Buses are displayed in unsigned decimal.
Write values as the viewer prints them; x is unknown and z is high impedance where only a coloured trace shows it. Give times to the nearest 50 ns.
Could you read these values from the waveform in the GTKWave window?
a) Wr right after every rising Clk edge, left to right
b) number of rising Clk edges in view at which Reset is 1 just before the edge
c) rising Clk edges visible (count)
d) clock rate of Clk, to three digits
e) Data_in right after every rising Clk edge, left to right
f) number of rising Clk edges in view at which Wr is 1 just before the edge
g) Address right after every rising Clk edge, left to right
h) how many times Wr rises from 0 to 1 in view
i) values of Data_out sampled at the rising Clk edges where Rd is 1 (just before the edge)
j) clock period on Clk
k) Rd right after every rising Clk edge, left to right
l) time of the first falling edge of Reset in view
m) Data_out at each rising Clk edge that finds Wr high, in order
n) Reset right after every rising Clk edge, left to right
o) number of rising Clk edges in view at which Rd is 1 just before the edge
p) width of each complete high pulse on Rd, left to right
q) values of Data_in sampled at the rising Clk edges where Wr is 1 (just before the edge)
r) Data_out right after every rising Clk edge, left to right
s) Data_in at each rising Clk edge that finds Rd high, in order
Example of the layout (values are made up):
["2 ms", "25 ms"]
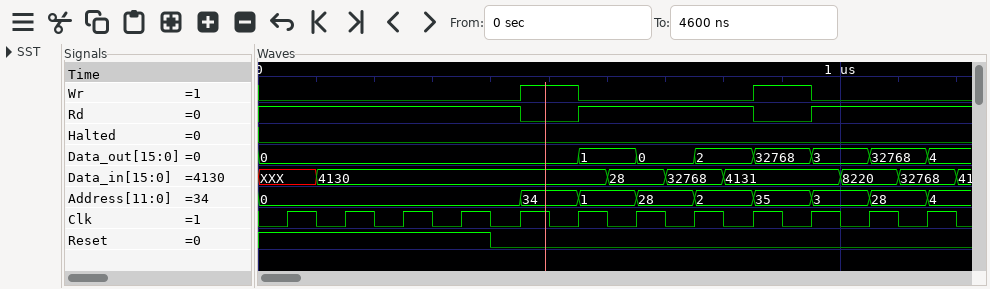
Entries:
["0 0 0 0 1 0 0 0 1 0 0 0", "4", "12", "10.0 MHz", "XXX, 4130, 4130, 4130, 4130, 4130, 28, 32768, 4131, 4131, 8220, 32768", "2", "0, 0, 0, 0, 34, 1, 28, 2, 35, 3, 28, 4", "2", "0, 0, 0, 0, 0, 1, 0, 2, 3, 32768", "100 ns", "1 1 1 1 0 1 1 1 0 1 1 1", "400 ns", "0, 32768", "1 1 1 1 0 0 0 0 0 0 0 0", "10", "300 ns", "4130, 4131", "0, 0, 0, 0, 0, 1, 0, 2, 32768, 3, 32768, 4", "XXX, 4130, 4130, 4130, 4130, 28, 32768, 4131, 8220, 32768"]
